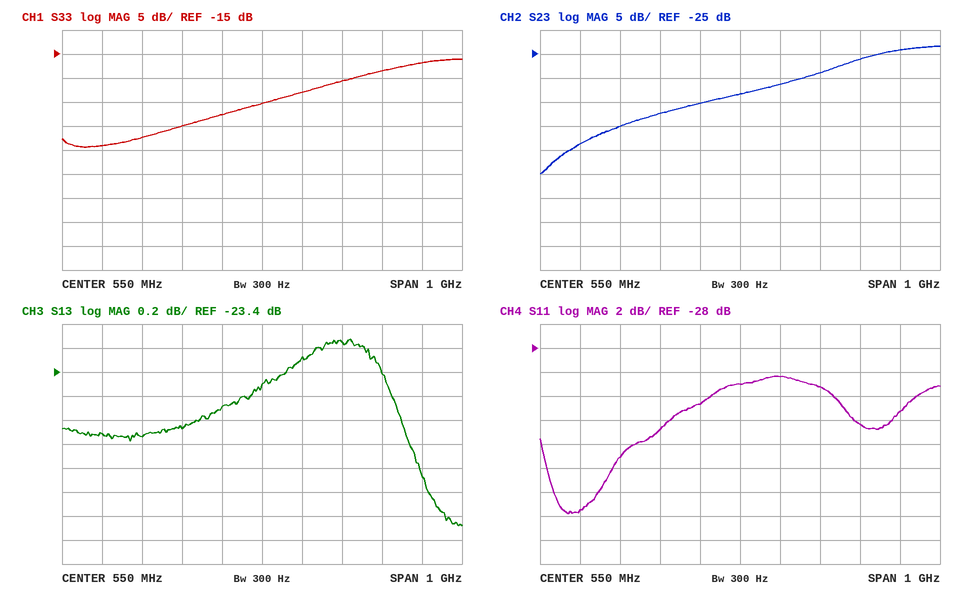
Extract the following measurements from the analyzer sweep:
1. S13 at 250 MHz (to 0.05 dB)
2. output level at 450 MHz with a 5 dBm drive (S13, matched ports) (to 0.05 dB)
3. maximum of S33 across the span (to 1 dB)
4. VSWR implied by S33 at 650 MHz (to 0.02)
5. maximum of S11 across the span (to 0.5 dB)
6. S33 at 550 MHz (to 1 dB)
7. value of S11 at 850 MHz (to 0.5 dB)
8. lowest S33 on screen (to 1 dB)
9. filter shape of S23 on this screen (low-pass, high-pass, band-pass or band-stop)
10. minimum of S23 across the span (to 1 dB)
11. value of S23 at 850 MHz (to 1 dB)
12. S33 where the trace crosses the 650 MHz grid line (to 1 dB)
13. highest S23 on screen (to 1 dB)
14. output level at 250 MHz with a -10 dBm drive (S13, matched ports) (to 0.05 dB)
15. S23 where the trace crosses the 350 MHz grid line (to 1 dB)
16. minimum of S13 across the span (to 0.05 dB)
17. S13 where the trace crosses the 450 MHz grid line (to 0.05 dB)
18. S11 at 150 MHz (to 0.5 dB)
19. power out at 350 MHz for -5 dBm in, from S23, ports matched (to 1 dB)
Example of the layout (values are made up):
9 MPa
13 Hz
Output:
-23.95 dB
-18.70 dBm
-16 dB
1.16
-30.5 dB
-25 dB
-34.5 dB
-34 dB
high-pass
-50 dB
-26 dB
-23 dB
-23 dB
-33.95 dBm
-37 dB
-24.70 dB
-23.70 dB
-41.5 dB
-42 dBm
